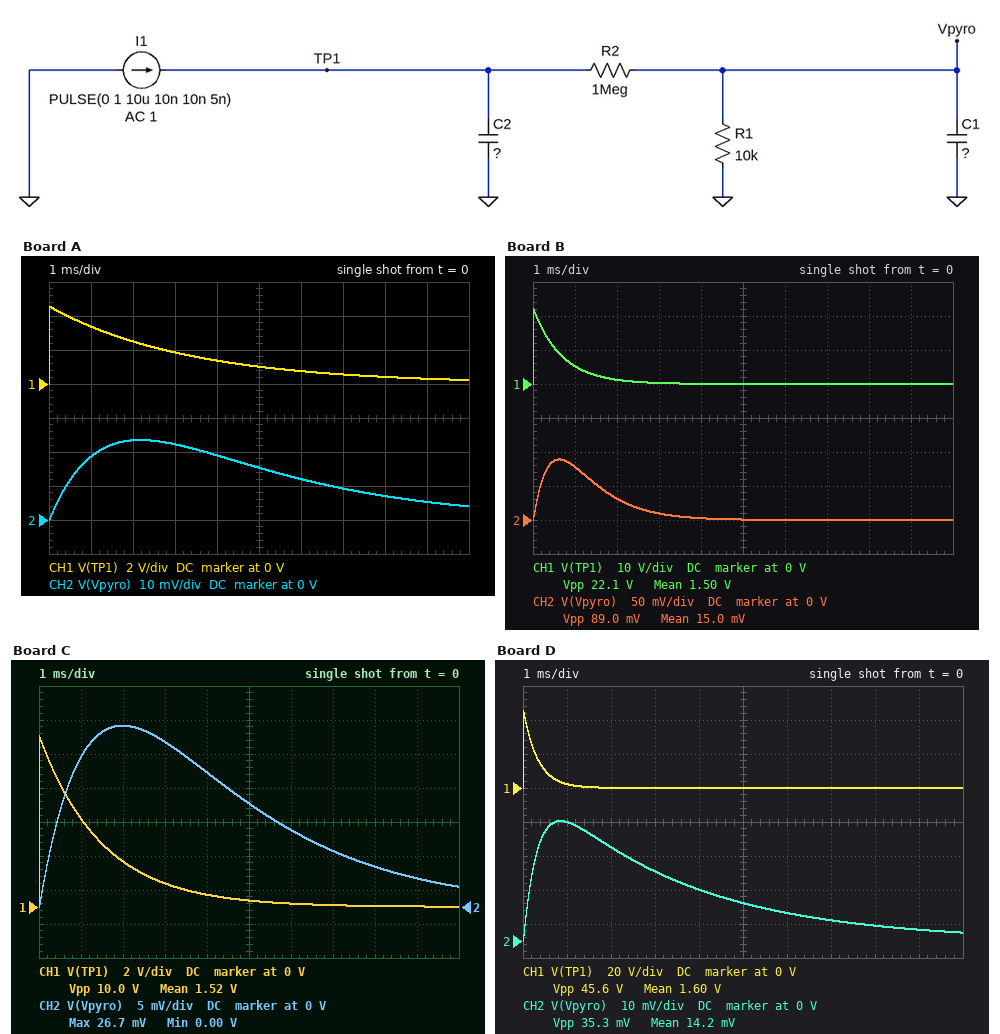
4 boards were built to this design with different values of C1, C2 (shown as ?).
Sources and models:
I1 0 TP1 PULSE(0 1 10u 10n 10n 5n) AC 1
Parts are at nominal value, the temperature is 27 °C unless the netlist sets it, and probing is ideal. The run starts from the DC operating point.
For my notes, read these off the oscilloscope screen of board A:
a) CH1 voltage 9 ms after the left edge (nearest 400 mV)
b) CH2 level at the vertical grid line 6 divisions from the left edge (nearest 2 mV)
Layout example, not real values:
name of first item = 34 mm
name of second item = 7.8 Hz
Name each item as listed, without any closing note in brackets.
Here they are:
CH1 voltage 9 ms after the left edge = 400 mV
CH2 level at the vertical grid line 6 divisions from the left edge = 12 mV
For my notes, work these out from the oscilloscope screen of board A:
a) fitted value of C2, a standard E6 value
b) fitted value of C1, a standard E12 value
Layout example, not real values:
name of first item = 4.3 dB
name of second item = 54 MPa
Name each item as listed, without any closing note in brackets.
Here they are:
fitted value of C2, a standard E6 value = 3.3 nF
fitted value of C1, a standard E12 value = 150 nF
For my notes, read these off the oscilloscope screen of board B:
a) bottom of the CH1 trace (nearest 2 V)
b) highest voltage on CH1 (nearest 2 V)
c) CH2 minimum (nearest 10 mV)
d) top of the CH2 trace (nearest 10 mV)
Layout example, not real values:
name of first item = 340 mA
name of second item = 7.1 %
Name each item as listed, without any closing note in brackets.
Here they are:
bottom of the CH1 trace = 0 V
highest voltage on CH1 = 22 V
CH2 minimum = 0 V
top of the CH2 trace = 90 mV
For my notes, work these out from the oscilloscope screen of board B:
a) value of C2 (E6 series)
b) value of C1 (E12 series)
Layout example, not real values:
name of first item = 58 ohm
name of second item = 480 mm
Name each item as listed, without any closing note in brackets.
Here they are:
value of C2 = 680 pF
value of C1 = 56 nF
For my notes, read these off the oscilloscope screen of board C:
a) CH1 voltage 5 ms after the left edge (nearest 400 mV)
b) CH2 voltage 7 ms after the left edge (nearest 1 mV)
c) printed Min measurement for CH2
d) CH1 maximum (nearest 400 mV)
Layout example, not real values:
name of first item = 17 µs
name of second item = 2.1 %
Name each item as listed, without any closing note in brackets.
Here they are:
CH1 voltage 5 ms after the left edge = 400 mV
CH2 voltage 7 ms after the left edge = 8 mV
printed Min measurement for CH2 = 0.00 V
CH1 maximum = 10.0 V
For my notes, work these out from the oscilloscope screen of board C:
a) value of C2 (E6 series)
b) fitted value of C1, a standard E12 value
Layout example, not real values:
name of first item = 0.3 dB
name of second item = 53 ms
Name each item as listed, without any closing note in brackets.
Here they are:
value of C2 = 1.5 nF
fitted value of C1, a standard E12 value = 270 nF
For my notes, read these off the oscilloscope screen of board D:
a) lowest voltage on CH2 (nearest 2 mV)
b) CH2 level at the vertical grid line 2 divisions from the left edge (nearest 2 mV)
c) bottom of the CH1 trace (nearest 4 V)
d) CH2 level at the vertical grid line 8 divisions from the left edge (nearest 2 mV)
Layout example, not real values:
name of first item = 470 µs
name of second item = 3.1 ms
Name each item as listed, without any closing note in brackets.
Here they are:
lowest voltage on CH2 = 0 V
CH2 level at the vertical grid line 2 divisions from the left edge = 28 mV
bottom of the CH1 trace = 0 V
CH2 level at the vertical grid line 8 divisions from the left edge = 4 mV
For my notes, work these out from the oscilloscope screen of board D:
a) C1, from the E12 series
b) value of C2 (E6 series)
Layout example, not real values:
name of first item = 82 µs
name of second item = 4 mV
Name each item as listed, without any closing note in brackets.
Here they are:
C1, from the E12 series = 330 nF
value of C2 = 330 pF
